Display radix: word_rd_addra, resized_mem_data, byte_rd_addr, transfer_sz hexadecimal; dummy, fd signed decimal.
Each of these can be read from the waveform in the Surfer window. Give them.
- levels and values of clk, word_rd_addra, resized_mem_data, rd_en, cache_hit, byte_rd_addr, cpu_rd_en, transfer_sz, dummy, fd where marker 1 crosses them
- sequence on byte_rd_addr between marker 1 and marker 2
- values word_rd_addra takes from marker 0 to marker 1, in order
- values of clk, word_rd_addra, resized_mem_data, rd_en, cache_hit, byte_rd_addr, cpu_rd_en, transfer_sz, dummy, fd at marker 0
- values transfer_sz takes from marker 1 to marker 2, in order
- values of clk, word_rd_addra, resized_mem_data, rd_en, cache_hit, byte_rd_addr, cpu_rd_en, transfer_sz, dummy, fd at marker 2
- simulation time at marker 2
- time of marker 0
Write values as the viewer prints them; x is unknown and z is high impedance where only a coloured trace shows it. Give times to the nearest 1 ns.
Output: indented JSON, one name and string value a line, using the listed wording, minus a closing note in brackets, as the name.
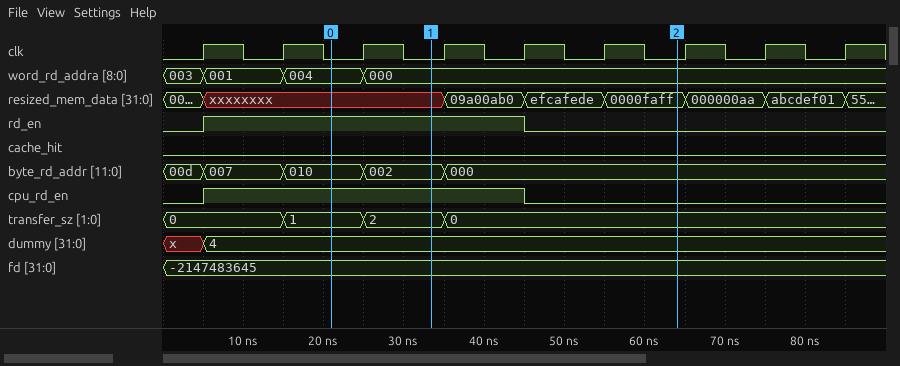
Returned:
{
  "levels and values of clk, word_rd_addra, resized_mem_data, rd_en, cache_hit, byte_rd_addr, cpu_rd_en, transfer_sz, dummy, fd where marker 1 crosses them": "clk=0, word_rd_addra=000, resized_mem_data=xxxxxxxx, rd_en=1, cache_hit=0, byte_rd_addr=002, cpu_rd_en=1, transfer_sz=2, dummy=4, fd=-2147483645",
  "sequence on byte_rd_addr between marker 1 and marker 2": "002, 000",
  "values word_rd_addra takes from marker 0 to marker 1, in order": "004, 000",
  "values of clk, word_rd_addra, resized_mem_data, rd_en, cache_hit, byte_rd_addr, cpu_rd_en, transfer_sz, dummy, fd at marker 0": "clk=0, word_rd_addra=004, resized_mem_data=xxxxxxxx, rd_en=1, cache_hit=0, byte_rd_addr=010, cpu_rd_en=1, transfer_sz=1, dummy=4, fd=-2147483645",
  "values transfer_sz takes from marker 1 to marker 2, in order": "2, 0",
  "values of clk, word_rd_addra, resized_mem_data, rd_en, cache_hit, byte_rd_addr, cpu_rd_en, transfer_sz, dummy, fd at marker 2": "clk=0, word_rd_addra=000, resized_mem_data=0000faff, rd_en=0, cache_hit=0, byte_rd_addr=000, cpu_rd_en=0, transfer_sz=0, dummy=4, fd=-2147483645",
  "simulation time at marker 2": "64 ns",
  "time of marker 0": "21 ns"
}
